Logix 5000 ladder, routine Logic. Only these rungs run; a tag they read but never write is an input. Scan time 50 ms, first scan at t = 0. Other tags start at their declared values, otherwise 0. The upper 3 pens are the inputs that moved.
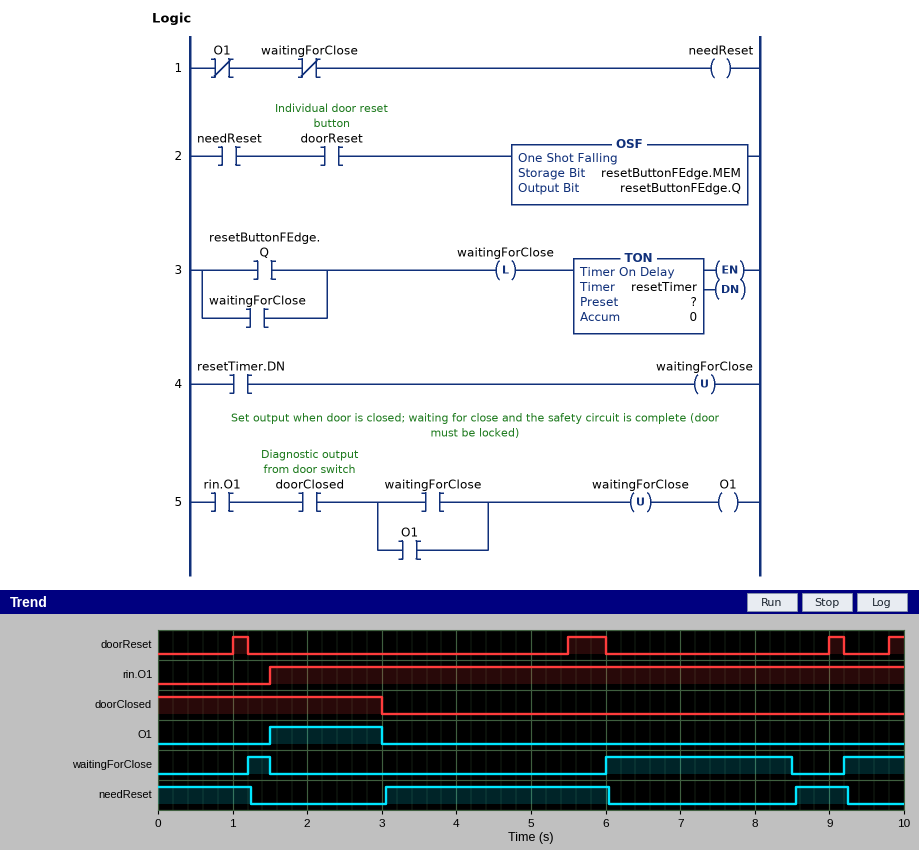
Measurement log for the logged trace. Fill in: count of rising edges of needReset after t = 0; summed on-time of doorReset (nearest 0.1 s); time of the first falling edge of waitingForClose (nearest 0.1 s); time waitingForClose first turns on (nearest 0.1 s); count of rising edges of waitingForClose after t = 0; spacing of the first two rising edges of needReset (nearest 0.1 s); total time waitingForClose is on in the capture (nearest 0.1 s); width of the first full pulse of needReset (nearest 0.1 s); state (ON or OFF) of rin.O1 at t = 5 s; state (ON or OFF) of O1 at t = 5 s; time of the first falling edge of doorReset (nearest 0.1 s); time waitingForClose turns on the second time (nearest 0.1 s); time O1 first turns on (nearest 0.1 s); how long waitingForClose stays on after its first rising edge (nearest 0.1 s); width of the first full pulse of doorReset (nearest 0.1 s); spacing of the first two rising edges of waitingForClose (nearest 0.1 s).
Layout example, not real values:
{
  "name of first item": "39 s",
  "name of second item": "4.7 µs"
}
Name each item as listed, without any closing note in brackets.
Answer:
{
  "count of rising edges of needReset after t = 0": "2",
  "summed on-time of doorReset": "1.1 s",
  "time of the first falling edge of waitingForClose": "1.5 s",
  "time waitingForClose first turns on": "1.2 s",
  "count of rising edges of waitingForClose after t = 0": "3",
  "spacing of the first two rising edges of needReset": "5.5 s",
  "total time waitingForClose is on in the capture": "3.6 s",
  "width of the first full pulse of needReset": "3.0 s",
  "state (ON or OFF) of rin.O1 at t = 5 s": "ON",
  "state (ON or OFF) of O1 at t = 5 s": "OFF",
  "time of the first falling edge of doorReset": "1.2 s",
  "time waitingForClose turns on the second time": "6.0 s",
  "time O1 first turns on": "1.5 s",
  "how long waitingForClose stays on after its first rising edge": "0.3 s",
  "width of the first full pulse of doorReset": "0.2 s",
  "spacing of the first two rising edges of waitingForClose": "4.8 s"
}
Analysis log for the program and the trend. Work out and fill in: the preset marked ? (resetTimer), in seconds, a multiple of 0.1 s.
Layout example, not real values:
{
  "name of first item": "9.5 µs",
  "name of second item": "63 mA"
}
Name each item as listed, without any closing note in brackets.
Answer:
{
  "the preset marked ? (resetTimer), in seconds, a multiple of 0.1 s": "2.5 s"
}
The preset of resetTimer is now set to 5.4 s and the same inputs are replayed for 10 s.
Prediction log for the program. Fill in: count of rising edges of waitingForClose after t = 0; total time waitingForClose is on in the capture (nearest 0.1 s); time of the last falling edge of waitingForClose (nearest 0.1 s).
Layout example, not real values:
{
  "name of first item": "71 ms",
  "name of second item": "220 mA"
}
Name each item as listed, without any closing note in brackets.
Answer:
{
  "count of rising edges of waitingForClose after t = 0": "2",
  "total time waitingForClose is on in the capture": "4.3 s",
  "time of the last falling edge of waitingForClose": "1.5 s"
}
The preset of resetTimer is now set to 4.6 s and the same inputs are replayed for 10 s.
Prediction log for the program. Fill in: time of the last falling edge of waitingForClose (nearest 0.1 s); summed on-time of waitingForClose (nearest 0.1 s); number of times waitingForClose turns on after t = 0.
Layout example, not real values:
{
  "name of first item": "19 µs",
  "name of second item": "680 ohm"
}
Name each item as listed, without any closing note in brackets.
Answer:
{
  "time of the last falling edge of waitingForClose": "1.5 s",
  "summed on-time of waitingForClose": "4.3 s",
  "number of times waitingForClose turns on after t = 0": "2"
}
